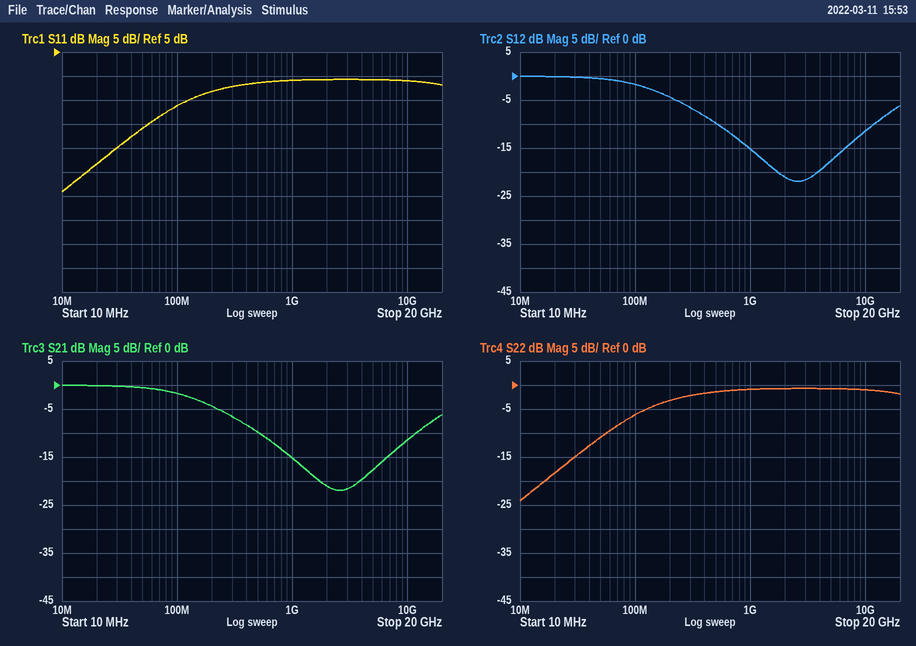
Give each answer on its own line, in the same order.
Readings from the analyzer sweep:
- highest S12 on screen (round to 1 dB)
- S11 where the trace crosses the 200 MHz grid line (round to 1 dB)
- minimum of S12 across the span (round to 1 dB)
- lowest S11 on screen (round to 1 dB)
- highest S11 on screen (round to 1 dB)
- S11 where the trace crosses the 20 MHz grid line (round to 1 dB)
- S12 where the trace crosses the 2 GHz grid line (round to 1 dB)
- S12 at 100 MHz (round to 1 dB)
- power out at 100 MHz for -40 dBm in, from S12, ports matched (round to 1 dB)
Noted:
0 dB
-3 dB
-22 dB
-24 dB
-1 dB
-18 dB
-21 dB
-2 dB
-42 dBm
